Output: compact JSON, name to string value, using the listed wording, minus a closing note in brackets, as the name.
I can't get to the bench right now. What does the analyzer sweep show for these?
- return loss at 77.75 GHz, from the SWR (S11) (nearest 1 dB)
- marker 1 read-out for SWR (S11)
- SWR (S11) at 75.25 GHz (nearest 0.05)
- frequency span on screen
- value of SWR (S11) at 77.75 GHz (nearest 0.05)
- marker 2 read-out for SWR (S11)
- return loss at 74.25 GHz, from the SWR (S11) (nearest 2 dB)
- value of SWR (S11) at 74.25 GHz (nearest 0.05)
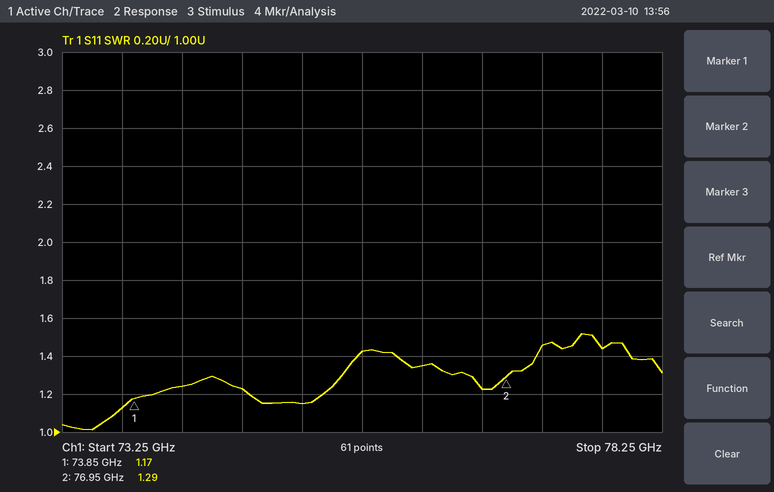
{"return loss at 77.75 GHz, from the SWR (S11)": "15 dB", "marker 1 read-out for SWR": "1.17", "SWR (S11) at 75.25 GHz": "1.15", "frequency span on screen": "5 GHz", "value of SWR (S11) at 77.75 GHz": "1.45", "marker 2 read-out for SWR": "1.29", "return loss at 74.25 GHz, from the SWR (S11)": "20 dB", "value of SWR (S11) at 74.25 GHz": "1.25"}
